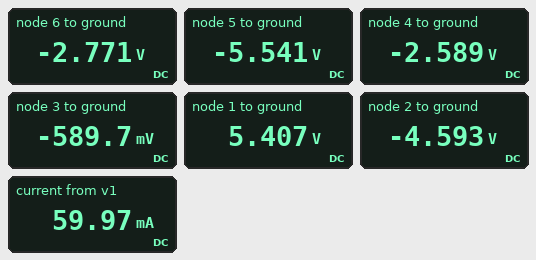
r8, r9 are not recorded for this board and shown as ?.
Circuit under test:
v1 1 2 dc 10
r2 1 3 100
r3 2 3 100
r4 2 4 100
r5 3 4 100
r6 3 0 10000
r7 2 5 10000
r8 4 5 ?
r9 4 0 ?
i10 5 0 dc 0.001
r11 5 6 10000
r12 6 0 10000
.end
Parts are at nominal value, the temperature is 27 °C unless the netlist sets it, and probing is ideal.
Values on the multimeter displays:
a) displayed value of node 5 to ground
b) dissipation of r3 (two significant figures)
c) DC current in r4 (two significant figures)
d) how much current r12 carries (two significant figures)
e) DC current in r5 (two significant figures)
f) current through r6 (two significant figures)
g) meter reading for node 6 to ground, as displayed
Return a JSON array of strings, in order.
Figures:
["-5.541 V", "160 mW", "20 mA", "280 µA", "20 mA", "59 µA", "-2.771 V"]
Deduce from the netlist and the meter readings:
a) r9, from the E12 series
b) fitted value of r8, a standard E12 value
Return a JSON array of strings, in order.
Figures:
["3.9 kΩ", "4.7 kΩ"]
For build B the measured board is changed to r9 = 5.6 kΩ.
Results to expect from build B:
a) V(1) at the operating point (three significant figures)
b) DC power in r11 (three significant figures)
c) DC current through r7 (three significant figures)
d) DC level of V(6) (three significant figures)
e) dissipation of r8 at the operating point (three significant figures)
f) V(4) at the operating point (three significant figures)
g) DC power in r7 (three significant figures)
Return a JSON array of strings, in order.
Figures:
["4.78 V", "925 µW", "86.4 µA", "-3.04 V", "1.75 mW", "-3.22 V", "74.7 µW"]
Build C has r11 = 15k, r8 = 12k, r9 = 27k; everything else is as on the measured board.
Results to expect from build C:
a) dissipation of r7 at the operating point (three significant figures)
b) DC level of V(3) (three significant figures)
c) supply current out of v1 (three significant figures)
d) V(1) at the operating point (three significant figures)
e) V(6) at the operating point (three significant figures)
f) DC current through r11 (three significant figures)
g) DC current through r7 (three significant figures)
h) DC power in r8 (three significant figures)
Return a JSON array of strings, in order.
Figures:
["545 µW", "-3.79 V", "59.9 mA", "2.19 V", "-4.06 V", "406 µA", "233 µA", "1.56 mW"]
